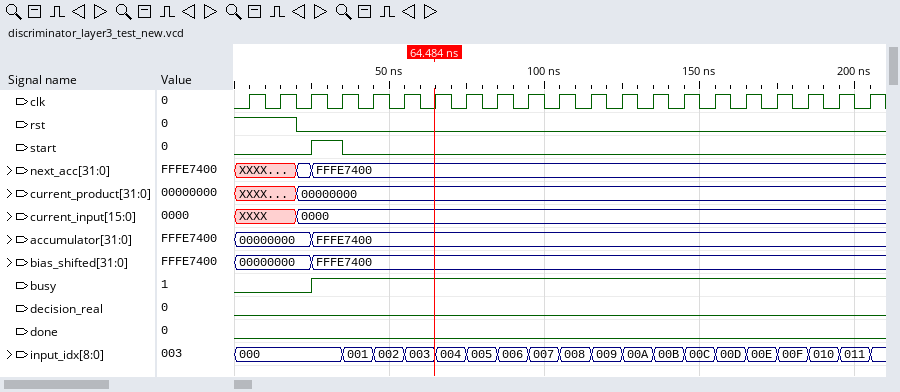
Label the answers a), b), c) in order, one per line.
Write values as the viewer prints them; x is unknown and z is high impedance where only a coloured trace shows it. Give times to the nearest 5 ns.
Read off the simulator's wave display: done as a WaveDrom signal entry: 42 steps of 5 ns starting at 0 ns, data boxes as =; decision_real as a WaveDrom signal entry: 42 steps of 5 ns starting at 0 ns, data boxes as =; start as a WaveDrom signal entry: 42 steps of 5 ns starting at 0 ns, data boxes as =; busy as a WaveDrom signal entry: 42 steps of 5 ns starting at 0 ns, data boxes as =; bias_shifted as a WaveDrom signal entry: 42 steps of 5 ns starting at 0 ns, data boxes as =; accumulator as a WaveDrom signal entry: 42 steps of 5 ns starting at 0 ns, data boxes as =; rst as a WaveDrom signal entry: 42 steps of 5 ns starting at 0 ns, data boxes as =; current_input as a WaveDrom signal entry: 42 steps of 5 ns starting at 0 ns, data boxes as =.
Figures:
a) {name: 'done', wave: '0.........................................'}
b) {name: 'decision_real', wave: '0.........................................'}
c) {name: 'start', wave: '0....1.0..................................'}
d) {name: 'busy', wave: '0....1....................................'}
e) {name: 'bias_shifted', wave: '=....=....................................', data: '00000000 FFFE7400'}
f) {name: 'accumulator', wave: '=....=....................................', data: '00000000 FFFE7400'}
g) {name: 'rst', wave: '1...0.....................................'}
h) {name: 'current_input', wave: 'x...=.....................................', data: '0000'}
